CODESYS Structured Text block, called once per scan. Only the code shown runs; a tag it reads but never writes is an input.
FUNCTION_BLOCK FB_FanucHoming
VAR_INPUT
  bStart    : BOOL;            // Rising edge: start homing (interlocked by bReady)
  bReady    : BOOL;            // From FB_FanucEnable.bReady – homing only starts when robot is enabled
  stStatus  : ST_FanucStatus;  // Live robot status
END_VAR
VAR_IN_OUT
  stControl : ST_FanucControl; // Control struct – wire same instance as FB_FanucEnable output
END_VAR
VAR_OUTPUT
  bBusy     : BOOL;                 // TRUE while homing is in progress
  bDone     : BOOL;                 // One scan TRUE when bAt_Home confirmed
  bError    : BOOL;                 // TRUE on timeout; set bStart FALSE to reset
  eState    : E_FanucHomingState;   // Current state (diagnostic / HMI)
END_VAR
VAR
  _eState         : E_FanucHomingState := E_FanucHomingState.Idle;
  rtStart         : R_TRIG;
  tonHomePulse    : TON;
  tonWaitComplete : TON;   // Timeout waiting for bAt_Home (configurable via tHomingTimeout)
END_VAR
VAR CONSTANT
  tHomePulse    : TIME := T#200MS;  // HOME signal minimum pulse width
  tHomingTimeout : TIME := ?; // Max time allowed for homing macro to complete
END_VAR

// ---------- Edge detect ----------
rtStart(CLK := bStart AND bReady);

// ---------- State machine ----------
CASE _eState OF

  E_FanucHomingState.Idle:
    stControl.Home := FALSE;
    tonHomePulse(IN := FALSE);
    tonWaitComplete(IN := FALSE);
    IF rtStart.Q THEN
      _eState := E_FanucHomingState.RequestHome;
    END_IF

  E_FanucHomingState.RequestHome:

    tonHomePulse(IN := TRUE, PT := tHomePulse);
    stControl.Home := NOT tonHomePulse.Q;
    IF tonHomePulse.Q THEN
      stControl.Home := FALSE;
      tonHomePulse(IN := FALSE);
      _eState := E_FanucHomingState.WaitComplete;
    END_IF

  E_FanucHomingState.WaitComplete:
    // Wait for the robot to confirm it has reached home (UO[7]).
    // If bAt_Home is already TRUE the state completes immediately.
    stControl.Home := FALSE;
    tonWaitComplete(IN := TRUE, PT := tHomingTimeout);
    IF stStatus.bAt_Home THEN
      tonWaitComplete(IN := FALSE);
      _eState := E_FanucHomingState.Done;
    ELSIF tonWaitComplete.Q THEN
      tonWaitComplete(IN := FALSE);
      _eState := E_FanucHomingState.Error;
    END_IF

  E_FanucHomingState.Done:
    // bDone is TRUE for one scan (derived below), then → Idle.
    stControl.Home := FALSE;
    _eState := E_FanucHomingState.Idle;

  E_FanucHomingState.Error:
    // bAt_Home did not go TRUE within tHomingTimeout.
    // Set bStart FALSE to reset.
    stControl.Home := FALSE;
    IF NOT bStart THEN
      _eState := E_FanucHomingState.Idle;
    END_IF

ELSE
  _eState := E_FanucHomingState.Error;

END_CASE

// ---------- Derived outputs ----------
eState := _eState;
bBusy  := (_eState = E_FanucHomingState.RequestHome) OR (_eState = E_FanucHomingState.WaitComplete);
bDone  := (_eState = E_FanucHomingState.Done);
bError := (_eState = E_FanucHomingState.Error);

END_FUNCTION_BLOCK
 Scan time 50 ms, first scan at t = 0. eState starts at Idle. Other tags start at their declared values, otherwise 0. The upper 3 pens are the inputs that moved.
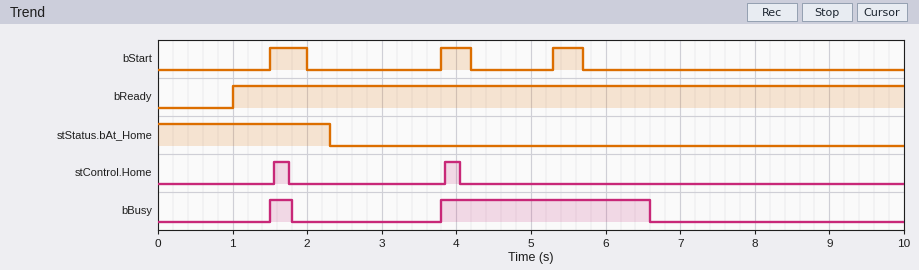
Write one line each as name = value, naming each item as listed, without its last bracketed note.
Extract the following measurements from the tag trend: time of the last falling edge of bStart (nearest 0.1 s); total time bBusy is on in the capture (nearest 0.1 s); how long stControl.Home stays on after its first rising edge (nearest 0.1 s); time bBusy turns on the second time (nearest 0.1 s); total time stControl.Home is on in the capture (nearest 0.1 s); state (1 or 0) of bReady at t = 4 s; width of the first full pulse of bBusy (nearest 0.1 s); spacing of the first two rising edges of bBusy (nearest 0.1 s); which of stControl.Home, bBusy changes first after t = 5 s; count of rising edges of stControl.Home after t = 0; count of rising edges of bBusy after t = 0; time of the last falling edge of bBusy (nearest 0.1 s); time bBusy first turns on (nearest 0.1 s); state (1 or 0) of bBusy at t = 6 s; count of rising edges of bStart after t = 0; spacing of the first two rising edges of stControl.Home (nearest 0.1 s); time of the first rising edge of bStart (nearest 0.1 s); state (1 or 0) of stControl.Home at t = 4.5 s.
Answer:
time of the last falling edge of bStart = 5.7 s
total time bBusy is on in the capture = 3.1 s
how long stControl.Home stays on after its first rising edge = 0.2 s
time bBusy turns on the second time = 3.8 s
total time stControl.Home is on in the capture = 0.4 s
state (1 or 0) of bReady at t = 4 s = 1
width of the first full pulse of bBusy = 0.3 s
spacing of the first two rising edges of bBusy = 2.3 s
which of stControl.Home, bBusy changes first after t = 5 s = bBusy
count of rising edges of stControl.Home after t = 0 = 2
count of rising edges of bBusy after t = 0 = 2
time of the last falling edge of bBusy = 6.6 s
time bBusy first turns on = 1.5 s
state (1 or 0) of bBusy at t = 6 s = 1
count of rising edges of bStart after t = 0 = 3
spacing of the first two rising edges of stControl.Home = 2.3 s
time of the first rising edge of bStart = 1.5 s
state (1 or 0) of stControl.Home at t = 4.5 s = 0
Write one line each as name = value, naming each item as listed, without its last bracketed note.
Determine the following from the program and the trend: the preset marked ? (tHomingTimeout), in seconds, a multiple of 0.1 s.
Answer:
the preset marked ? (tHomingTimeout), in seconds, a multiple of 0.1 s = 2.5 s
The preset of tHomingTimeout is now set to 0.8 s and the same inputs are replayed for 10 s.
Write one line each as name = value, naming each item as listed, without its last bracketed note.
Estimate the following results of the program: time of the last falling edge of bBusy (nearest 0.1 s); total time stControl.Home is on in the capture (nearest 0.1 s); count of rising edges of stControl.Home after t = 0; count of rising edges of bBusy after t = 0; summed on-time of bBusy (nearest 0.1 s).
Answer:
time of the last falling edge of bBusy = 6.4 s
total time stControl.Home is on in the capture = 0.6 s
count of rising edges of stControl.Home after t = 0 = 3
count of rising edges of bBusy after t = 0 = 3
summed on-time of bBusy = 2.5 s
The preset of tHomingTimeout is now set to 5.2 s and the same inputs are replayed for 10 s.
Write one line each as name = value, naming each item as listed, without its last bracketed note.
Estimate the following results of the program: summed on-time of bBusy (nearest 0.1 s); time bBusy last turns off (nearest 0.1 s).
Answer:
summed on-time of bBusy = 5.8 s
time bBusy last turns off = 9.3 s
